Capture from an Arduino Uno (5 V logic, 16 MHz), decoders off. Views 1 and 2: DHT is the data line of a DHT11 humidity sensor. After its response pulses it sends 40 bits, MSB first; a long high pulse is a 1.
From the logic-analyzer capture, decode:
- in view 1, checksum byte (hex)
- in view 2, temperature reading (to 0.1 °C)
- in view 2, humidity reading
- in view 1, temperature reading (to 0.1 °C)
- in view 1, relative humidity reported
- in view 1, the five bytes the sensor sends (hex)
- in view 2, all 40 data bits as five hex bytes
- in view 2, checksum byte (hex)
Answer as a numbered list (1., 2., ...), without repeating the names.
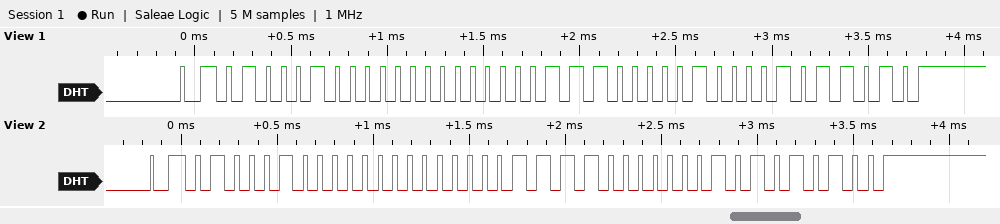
1. 0x5A
2. 15.1 °C
3. 68 %
4. 14.8 °C
5. 68 %
6. 44 00 0E 08 5A
7. 44 00 0F 01 54
8. 0x54
